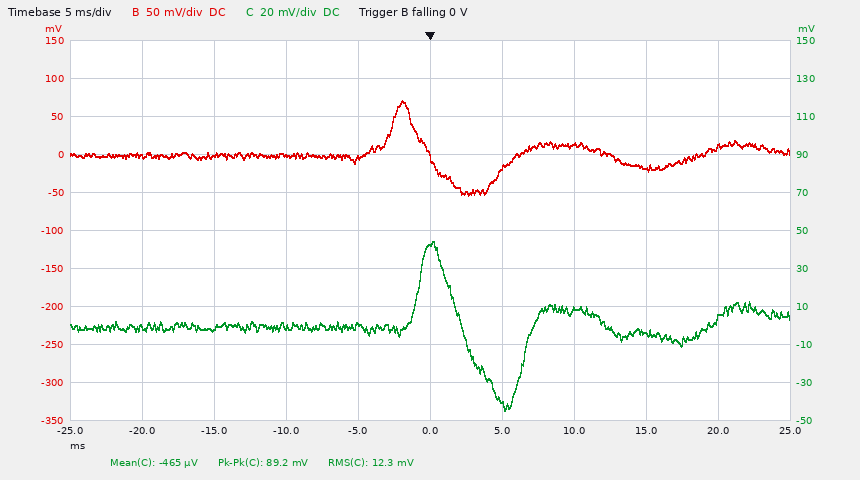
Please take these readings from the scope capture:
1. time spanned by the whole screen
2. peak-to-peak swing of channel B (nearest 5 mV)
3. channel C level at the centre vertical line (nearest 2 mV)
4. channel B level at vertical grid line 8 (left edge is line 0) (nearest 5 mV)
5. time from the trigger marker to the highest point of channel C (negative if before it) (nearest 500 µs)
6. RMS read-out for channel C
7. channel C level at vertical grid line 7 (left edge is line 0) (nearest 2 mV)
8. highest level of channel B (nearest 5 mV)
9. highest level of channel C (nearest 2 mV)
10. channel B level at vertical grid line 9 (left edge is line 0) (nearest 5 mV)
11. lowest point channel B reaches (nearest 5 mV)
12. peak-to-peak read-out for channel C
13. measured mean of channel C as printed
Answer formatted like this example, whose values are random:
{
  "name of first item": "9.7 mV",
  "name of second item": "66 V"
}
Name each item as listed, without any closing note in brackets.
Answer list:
{
  "time spanned by the whole screen": "50 ms",
  "peak-to-peak swing of channel B": "125 mV",
  "channel C level at the centre vertical line": "42 mV",
  "channel B level at vertical grid line 8 (left edge is line 0)": "-20 mV",
  "time from the trigger marker to the highest point of channel C (negative if before it)": "0.0 ms",
  "RMS read-out for channel C": "12.3 mV",
  "channel C level at vertical grid line 7 (left edge is line 0)": "8 mV",
  "highest level of channel B": "70 mV",
  "highest level of channel C": "44 mV",
  "channel B level at vertical grid line 9 (left edge is line 0)": "10 mV",
  "lowest point channel B reaches": "-55 mV",
  "peak-to-peak read-out for channel C": "89.2 mV",
  "measured mean of channel C as printed": "-465 µV"
}
